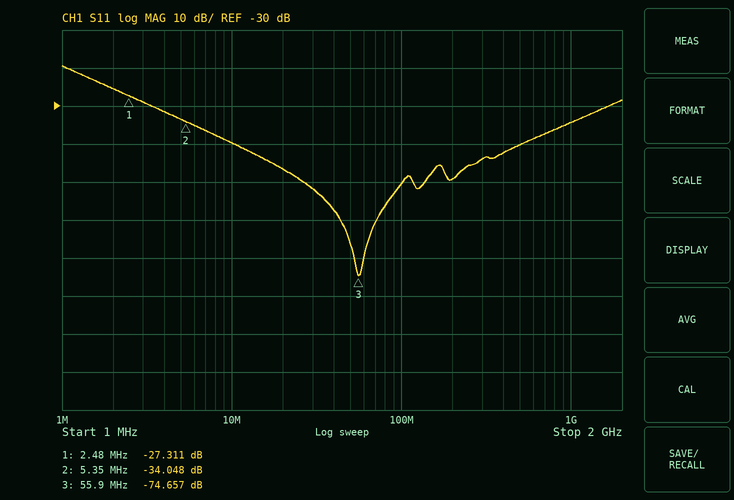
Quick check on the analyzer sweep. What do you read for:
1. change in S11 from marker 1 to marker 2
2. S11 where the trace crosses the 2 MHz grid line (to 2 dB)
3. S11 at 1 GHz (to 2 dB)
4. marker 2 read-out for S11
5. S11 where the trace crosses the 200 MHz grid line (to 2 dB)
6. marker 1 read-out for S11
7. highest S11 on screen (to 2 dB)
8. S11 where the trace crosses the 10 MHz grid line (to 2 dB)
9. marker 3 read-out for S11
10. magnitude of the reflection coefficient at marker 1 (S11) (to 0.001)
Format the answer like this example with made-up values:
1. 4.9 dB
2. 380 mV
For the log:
1. -6.737 dB
2. -26 dB
3. -34 dB
4. -34.048 dB
5. -50 dB
6. -27.311 dB
7. -20 dB
8. -40 dB
9. -74.657 dB
10. 0.043
